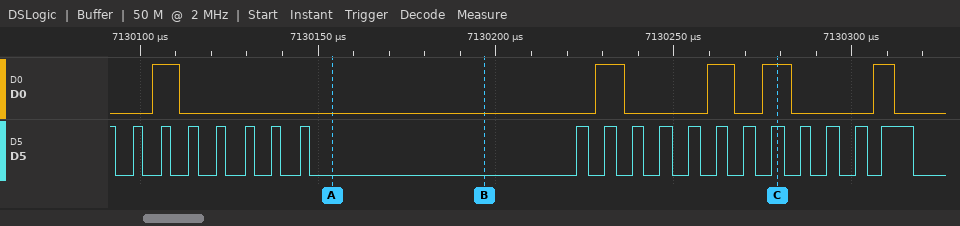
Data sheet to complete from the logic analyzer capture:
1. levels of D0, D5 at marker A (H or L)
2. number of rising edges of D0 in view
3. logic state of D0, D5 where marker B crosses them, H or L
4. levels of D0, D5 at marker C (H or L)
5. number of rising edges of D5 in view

D0=L, D5=L
5
D0=L, D5=L
D0=H, D5=H
19
